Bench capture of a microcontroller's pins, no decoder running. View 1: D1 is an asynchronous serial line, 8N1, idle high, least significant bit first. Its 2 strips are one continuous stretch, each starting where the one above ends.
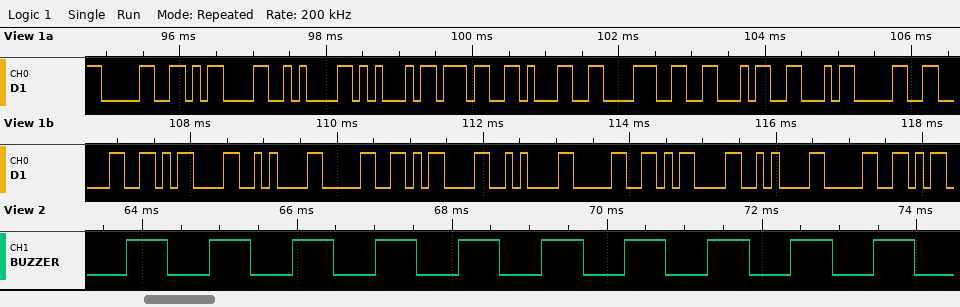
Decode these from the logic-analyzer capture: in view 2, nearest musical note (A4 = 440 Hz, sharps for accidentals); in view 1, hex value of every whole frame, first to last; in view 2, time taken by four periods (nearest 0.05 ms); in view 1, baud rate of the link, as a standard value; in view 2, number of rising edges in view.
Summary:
A#5
0x30 0x0D 0x0A 0x45 0x37 0x31 0x38 0x46 0x46 0x30 0x30 0x0D 0x0A 0x30 0x0D 0x0A 0x30 0x0D 0x0A 0x30
4.30 ms
9600 baud
10
